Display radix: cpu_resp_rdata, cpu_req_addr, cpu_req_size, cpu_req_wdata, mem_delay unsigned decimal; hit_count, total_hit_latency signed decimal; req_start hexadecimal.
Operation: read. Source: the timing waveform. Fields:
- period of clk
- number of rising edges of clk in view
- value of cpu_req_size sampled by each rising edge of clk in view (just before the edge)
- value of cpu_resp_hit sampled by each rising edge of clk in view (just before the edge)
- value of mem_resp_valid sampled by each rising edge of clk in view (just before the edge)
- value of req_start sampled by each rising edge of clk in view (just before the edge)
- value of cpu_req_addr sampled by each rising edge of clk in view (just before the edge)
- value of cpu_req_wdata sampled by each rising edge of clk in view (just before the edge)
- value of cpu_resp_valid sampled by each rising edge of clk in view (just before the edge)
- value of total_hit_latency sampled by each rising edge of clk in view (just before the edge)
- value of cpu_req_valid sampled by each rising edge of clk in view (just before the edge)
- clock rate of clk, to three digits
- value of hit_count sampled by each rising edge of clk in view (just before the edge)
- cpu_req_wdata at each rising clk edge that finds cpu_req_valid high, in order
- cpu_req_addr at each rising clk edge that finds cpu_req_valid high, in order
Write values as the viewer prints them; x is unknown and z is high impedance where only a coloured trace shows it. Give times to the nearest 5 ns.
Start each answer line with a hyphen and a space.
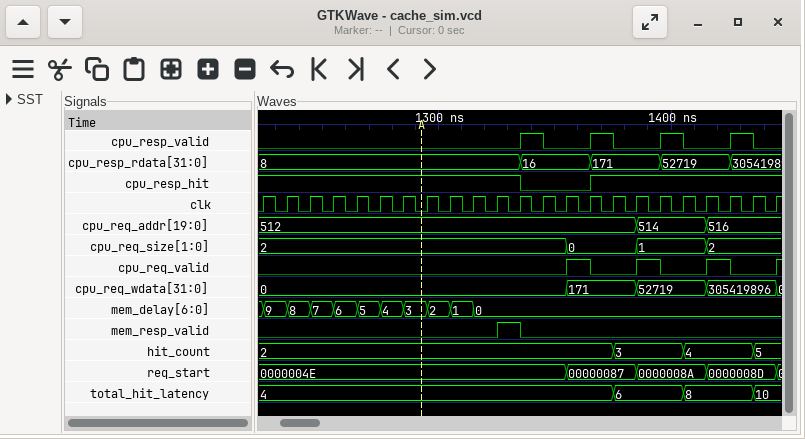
- 10 ns
- 23
- 2, 2, 2, 2, 2, 2, 2, 2, 2, 2, 2, 2, 2, 2, 0, 0, 0, 1, 1, 1, 2, 2, 2
- 1 1 1 1 1 1 1 1 1 1 1 1 0 0 0 1 1 1 1 1 1 1 1
- 0 0 0 0 0 0 0 0 0 0 0 1 0 0 0 0 0 0 0 0 0 0 0
- 0000004E, 0000004E, 0000004E, 0000004E, 0000004E, 0000004E, 0000004E, 0000004E, 0000004E, 0000004E, 0000004E, 0000004E, 0000004E, 0000004E, 00000087, 00000087, 00000087, 0000008A, 0000008A, 0000008A, 0000008D, 0000008D, 0000008D
- 512, 512, 512, 512, 512, 512, 512, 512, 512, 512, 512, 512, 512, 512, 512, 512, 512, 514, 514, 514, 516, 516, 516
- 0, 0, 0, 0, 0, 0, 0, 0, 0, 0, 0, 0, 0, 0, 171, 171, 171, 52719, 52719, 52719, 305419896, 305419896, 305419896
- 0 0 0 0 0 0 0 0 0 0 0 0 1 0 0 1 0 0 1 0 0 1 0
- 4, 4, 4, 4, 4, 4, 4, 4, 4, 4, 4, 4, 4, 4, 4, 4, 6, 6, 6, 8, 8, 8, 10
- 0 0 0 0 0 0 0 0 0 0 0 0 0 0 1 0 0 1 0 0 1 0 0
- 100 MHz
- 2, 2, 2, 2, 2, 2, 2, 2, 2, 2, 2, 2, 2, 2, 2, 2, 3, 3, 3, 4, 4, 4, 5
- 171, 52719, 305419896
- 512, 514, 516
